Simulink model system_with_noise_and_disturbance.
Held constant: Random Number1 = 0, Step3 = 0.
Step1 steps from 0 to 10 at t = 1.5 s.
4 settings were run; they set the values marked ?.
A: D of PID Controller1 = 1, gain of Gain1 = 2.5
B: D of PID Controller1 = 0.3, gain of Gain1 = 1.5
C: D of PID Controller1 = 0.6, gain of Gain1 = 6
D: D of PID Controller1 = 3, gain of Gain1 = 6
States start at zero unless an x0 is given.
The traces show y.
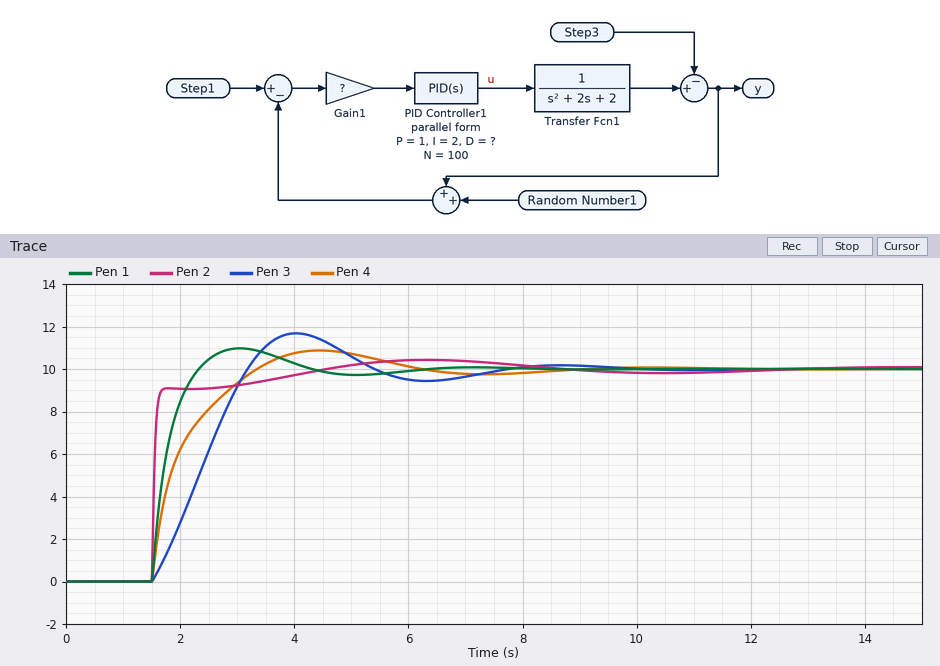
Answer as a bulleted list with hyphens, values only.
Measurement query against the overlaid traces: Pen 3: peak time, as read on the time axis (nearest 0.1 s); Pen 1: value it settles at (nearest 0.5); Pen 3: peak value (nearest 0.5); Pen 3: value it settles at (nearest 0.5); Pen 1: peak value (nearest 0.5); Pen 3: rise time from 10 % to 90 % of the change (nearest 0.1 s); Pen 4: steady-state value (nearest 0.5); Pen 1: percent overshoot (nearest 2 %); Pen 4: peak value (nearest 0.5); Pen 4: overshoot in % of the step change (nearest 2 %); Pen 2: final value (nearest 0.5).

- 4.0 s
- 10.0
- 11.5
- 10.0
- 11.0
- 1.3 s
- 10.0
- 10 %
- 11.0
- 8 %
- 10.0
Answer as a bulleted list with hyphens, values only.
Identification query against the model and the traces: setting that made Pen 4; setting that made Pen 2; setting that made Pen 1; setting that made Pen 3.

- A
- D
- C
- B
